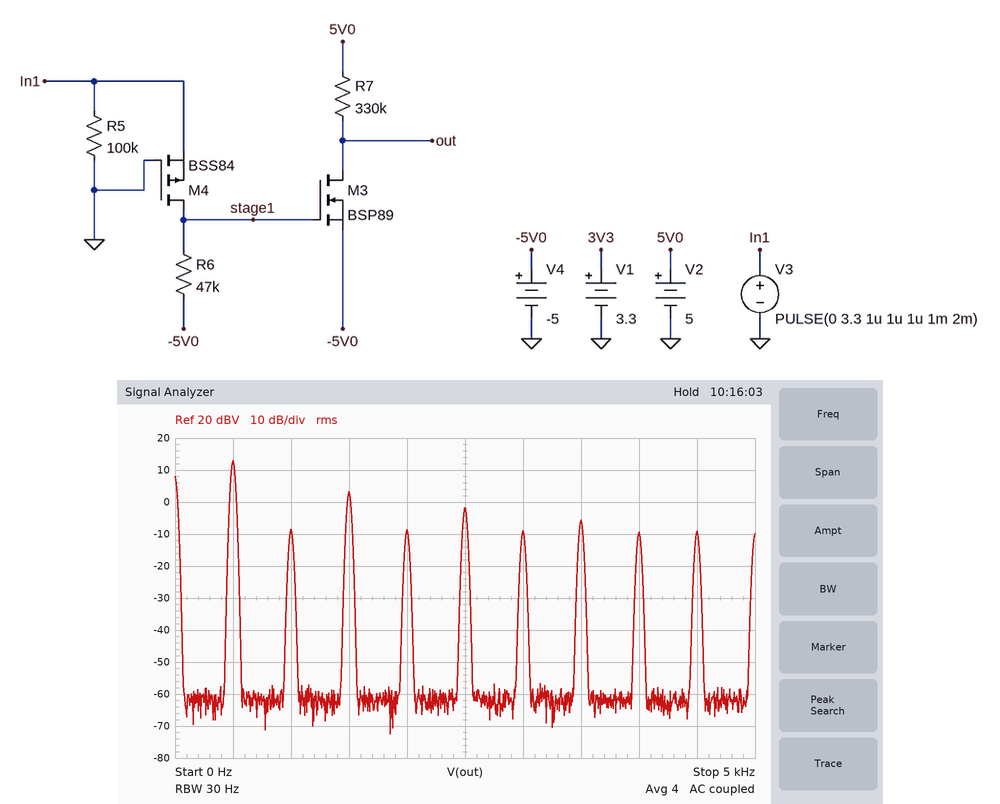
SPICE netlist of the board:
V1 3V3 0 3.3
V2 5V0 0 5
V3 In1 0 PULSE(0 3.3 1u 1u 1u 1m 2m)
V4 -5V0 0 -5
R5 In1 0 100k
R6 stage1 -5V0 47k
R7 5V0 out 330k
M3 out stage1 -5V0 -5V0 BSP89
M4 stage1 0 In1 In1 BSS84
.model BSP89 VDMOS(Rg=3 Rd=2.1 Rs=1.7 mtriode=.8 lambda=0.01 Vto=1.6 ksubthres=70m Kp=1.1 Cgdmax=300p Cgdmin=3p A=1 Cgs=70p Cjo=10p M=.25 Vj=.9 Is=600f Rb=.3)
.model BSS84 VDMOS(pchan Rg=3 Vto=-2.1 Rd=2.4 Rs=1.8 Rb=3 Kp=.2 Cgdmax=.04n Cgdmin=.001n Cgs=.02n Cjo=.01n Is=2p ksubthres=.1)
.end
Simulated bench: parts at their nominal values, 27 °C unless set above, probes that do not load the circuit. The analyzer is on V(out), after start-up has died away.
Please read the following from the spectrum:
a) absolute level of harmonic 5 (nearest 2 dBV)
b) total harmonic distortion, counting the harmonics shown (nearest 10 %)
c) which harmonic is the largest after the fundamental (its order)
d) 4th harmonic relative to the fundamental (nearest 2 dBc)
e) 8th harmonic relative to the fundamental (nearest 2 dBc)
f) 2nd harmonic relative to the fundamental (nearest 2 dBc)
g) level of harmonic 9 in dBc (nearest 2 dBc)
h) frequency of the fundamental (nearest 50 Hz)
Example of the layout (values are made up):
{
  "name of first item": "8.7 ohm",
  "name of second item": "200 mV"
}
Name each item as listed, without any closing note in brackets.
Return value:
{
  "absolute level of harmonic 5": "-2 dBV",
  "total harmonic distortion, counting the harmonics shown": "40 %",
  "which harmonic is the largest after the fundamental": "3",
  "4th harmonic relative to the fundamental": "-22 dBc",
  "8th harmonic relative to the fundamental": "-22 dBc",
  "2nd harmonic relative to the fundamental": "-22 dBc",
  "level of harmonic 9 in dBc": "-22 dBc",
  "frequency of the fundamental": "500 Hz"
}
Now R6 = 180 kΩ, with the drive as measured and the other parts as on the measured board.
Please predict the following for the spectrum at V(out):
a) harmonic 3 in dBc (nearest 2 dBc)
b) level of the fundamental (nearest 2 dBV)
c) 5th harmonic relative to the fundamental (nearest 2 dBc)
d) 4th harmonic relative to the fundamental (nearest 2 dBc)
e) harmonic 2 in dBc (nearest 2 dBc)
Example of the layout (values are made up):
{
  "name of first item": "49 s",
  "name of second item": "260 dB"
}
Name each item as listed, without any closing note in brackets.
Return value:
{
  "harmonic 3 in dBc": "-12 dBc",
  "level of the fundamental": "12 dBV",
  "5th harmonic relative to the fundamental": "-26 dBc",
  "4th harmonic relative to the fundamental": "-14 dBc",
  "harmonic 2 in dBc": "-12 dBc"
}
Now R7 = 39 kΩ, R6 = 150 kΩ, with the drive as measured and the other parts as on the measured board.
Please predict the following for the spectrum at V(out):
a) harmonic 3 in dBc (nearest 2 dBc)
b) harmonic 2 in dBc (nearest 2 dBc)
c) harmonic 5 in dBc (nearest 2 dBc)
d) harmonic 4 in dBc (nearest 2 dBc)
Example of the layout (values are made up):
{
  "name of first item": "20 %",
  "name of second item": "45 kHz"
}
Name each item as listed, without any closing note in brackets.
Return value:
{
  "harmonic 3 in dBc": "-12 dBc",
  "harmonic 2 in dBc": "-14 dBc",
  "harmonic 5 in dBc": "-20 dBc",
  "harmonic 4 in dBc": "-14 dBc"
}
